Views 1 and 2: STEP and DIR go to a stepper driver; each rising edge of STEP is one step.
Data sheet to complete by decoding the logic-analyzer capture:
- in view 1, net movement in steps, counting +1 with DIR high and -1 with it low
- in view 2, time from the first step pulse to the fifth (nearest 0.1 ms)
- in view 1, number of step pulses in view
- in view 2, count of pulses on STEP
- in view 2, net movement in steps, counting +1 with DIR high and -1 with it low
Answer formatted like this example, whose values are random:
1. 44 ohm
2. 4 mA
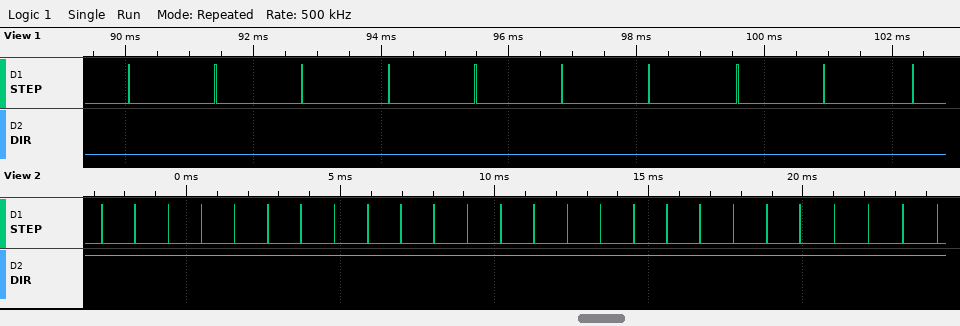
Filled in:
1. -10
2. 4.3 ms
3. 10
4. 26
5. +26
